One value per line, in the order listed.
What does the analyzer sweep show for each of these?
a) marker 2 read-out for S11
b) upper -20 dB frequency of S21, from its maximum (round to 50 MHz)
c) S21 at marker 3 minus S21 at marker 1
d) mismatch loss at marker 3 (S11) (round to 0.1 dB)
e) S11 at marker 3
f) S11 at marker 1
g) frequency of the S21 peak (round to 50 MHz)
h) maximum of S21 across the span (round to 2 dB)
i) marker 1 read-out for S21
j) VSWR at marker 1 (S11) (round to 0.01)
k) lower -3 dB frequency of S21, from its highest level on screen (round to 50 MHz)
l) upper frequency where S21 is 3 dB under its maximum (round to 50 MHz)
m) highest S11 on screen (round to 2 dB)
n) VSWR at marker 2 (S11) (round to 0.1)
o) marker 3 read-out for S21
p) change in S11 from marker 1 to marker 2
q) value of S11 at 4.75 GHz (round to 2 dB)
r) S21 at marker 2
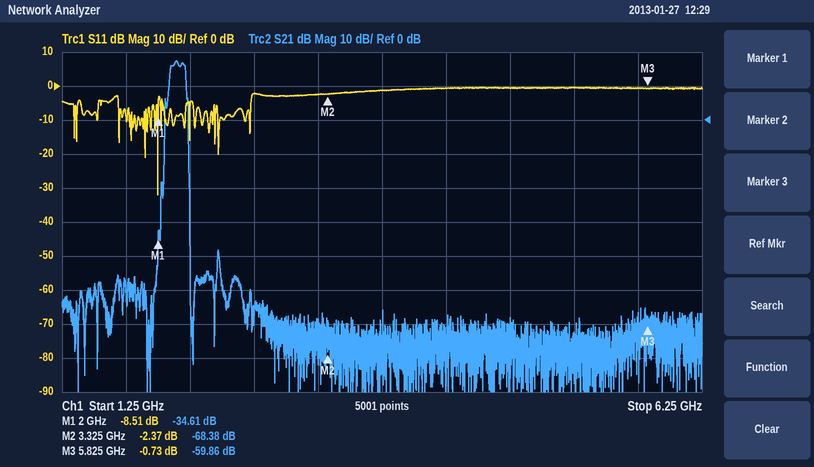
-2.37 dB
2.25 GHz
-25.25 dB
8.1 dB
-0.73 dB
-8.51 dB
2.15 GHz
18 dB
-34.61 dB
2.20
2.10 GHz
2.20 GHz
0 dB
7.4
-59.86 dB
6.14 dB
0 dB
-68.38 dB
